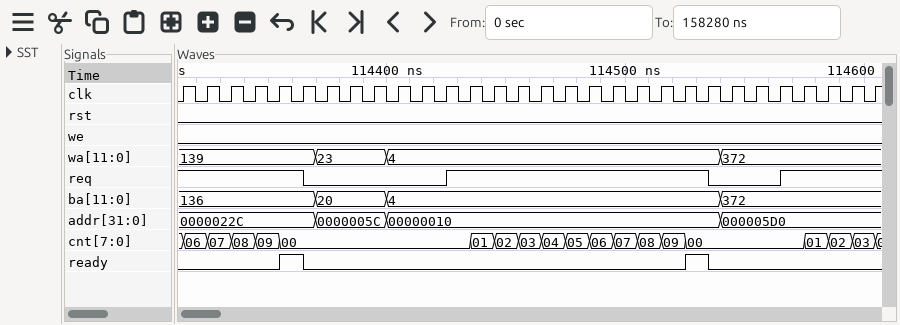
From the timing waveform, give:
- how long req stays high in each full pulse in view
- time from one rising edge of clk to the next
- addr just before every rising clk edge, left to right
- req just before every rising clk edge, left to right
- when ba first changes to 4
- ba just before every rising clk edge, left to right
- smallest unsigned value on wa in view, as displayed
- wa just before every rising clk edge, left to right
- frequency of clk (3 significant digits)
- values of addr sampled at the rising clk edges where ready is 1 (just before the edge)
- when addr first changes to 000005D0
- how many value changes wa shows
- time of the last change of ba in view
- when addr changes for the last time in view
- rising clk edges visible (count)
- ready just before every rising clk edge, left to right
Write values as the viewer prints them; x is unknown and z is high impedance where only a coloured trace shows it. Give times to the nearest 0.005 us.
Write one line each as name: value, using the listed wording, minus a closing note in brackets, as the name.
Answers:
how long req stays high in each full pulse in view: 0.11 us
time from one rising edge of clk to the next: 0.01 us
addr just before every rising clk edge, left to right: 0000022C, 0000022C, 0000022C, 0000022C, 0000022C, 0000022C, 0000005C, 0000005C, 0000005C, 00000010, 00000010, 00000010, 00000010, 00000010, 00000010, 00000010, 00000010, 00000010, 00000010, 00000010, 00000010, 00000010, 00000010, 000005D0, 000005D0, 000005D0, 000005D0, 000005D0, 000005D0, 000005D0
req just before every rising clk edge, left to right: 1 1 1 1 1 1 0 0 0 0 0 0 1 1 1 1 1 1 1 1 1 1 1 0 0 0 1 1 1 1
when ba first changes to 4: 114.4 us
ba just before every rising clk edge, left to right: 136, 136, 136, 136, 136, 136, 20, 20, 20, 4, 4, 4, 4, 4, 4, 4, 4, 4, 4, 4, 4, 4, 4, 372, 372, 372, 372, 372, 372, 372
smallest unsigned value on wa in view, as displayed: 4
wa just before every rising clk edge, left to right: 139, 139, 139, 139, 139, 139, 23, 23, 23, 4, 4, 4, 4, 4, 4, 4, 4, 4, 4, 4, 4, 4, 4, 372, 372, 372, 372, 372, 372, 372
frequency of clk: 100 MHz
values of addr sampled at the rising clk edges where ready is 1: 0000022C, 00000010
when addr first changes to 000005D0: 114.54 us
how many value changes wa shows: 3
time of the last change of ba in view: 114.54 us
when addr changes for the last time in view: 114.54 us
rising clk edges visible: 30
ready just before every rising clk edge, left to right: 0 0 0 0 0 1 0 0 0 0 0 0 0 0 0 0 0 0 0 0 0 0 1 0 0 0 0 0 0 0
